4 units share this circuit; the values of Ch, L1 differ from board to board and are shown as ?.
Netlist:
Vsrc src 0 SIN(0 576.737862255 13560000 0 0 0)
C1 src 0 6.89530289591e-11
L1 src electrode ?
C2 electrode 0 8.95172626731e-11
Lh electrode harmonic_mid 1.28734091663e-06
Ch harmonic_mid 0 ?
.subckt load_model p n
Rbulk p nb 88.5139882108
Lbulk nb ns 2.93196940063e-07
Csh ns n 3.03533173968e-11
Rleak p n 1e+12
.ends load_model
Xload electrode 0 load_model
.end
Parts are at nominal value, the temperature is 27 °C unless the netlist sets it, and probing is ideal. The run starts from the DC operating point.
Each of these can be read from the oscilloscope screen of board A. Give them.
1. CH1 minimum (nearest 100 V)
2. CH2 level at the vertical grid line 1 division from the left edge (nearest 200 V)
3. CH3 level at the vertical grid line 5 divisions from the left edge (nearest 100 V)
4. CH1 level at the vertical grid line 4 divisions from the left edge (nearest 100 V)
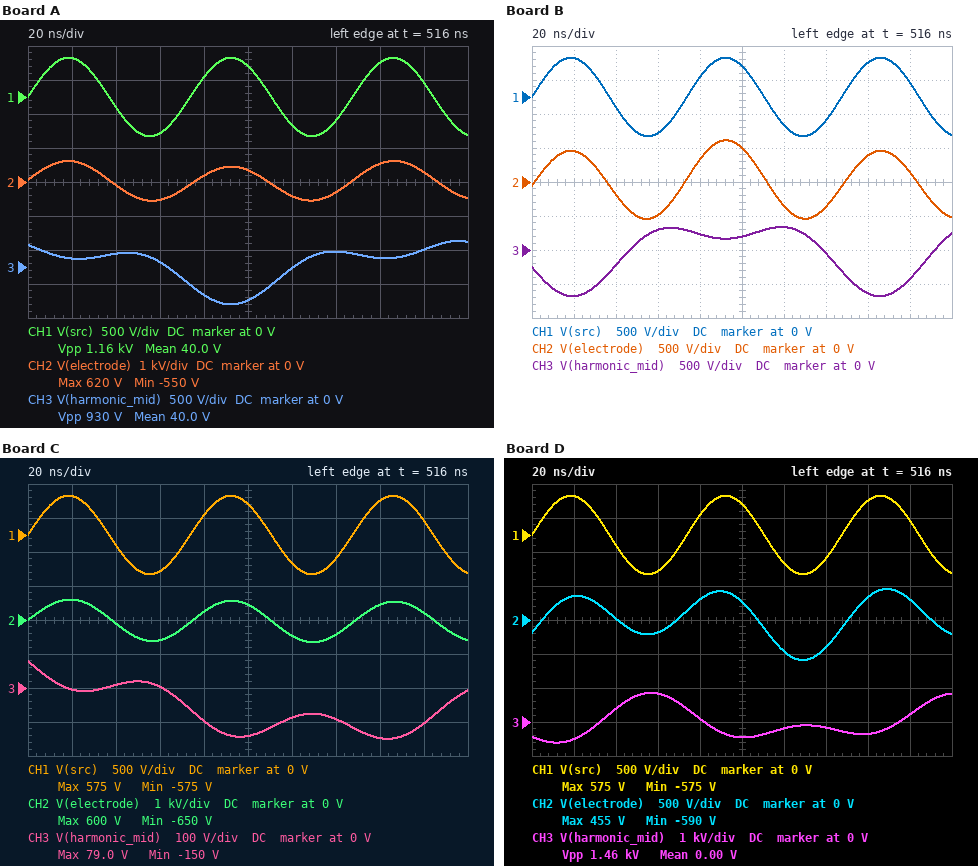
-600 V
600 V
-500 V
300 V
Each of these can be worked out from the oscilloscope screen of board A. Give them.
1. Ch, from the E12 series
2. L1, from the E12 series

390 pF
390 nH
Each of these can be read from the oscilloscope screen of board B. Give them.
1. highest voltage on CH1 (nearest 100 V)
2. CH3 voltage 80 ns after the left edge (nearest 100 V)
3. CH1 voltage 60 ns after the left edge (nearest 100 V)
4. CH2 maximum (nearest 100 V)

600 V
200 V
-500 V
600 V
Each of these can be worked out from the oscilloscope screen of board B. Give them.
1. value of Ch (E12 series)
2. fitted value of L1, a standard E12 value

330 pF
270 nH
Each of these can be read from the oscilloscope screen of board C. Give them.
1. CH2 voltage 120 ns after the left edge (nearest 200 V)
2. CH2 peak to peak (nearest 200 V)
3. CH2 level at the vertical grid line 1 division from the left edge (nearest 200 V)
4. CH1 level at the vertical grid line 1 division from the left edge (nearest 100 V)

-400 V
1.2 kV
600 V
600 V
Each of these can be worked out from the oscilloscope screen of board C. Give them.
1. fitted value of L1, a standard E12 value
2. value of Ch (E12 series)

1 µH
1.5 nF
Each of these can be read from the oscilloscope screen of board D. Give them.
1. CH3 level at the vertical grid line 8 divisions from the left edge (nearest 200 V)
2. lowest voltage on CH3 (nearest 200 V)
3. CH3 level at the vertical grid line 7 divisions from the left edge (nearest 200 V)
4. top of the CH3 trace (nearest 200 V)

-400 V
-600 V
-200 V
800 V
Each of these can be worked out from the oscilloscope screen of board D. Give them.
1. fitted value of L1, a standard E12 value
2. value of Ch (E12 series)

680 nH
220 pF
